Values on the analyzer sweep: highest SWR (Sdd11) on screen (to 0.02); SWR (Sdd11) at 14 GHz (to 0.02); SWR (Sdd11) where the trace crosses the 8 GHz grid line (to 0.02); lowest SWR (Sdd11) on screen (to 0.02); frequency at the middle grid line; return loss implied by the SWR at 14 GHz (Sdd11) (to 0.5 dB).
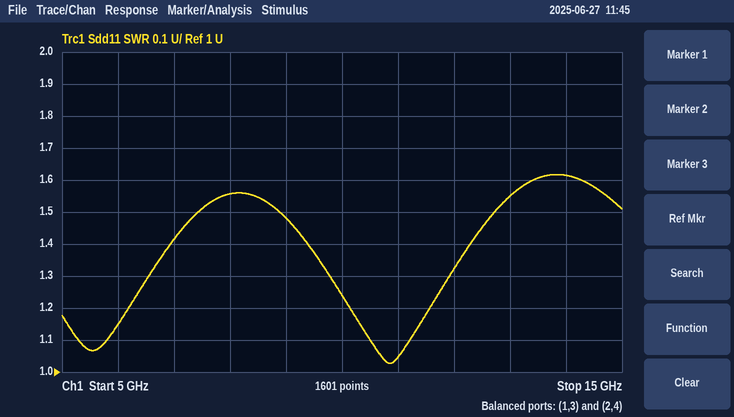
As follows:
1.62
1.62
1.56
1.02
10 GHz
12.5 dB
